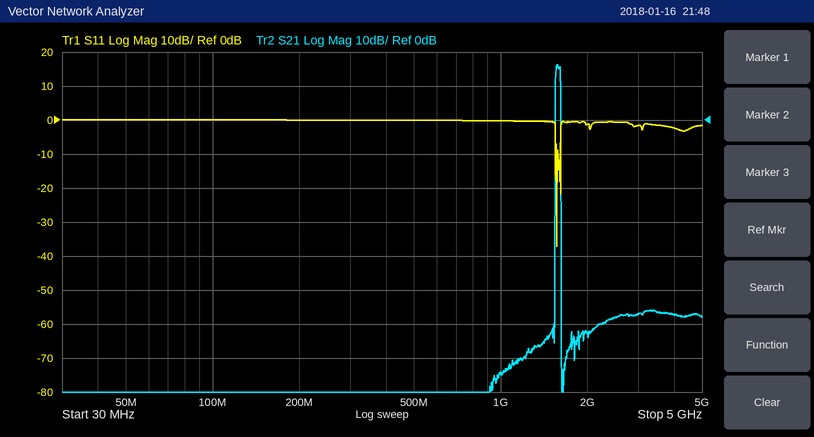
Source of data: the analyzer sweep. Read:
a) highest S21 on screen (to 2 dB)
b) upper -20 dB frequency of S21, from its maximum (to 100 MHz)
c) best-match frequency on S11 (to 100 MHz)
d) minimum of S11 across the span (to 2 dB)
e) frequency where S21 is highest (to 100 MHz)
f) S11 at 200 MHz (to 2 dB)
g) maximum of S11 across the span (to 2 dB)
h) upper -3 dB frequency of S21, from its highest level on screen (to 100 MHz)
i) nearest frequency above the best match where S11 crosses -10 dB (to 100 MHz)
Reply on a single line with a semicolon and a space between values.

16 dB; 1.6 GHz; 1.6 GHz; -38 dB; 1.6 GHz; 0 dB; 0 dB; 1.6 GHz; 1.6 GHz
